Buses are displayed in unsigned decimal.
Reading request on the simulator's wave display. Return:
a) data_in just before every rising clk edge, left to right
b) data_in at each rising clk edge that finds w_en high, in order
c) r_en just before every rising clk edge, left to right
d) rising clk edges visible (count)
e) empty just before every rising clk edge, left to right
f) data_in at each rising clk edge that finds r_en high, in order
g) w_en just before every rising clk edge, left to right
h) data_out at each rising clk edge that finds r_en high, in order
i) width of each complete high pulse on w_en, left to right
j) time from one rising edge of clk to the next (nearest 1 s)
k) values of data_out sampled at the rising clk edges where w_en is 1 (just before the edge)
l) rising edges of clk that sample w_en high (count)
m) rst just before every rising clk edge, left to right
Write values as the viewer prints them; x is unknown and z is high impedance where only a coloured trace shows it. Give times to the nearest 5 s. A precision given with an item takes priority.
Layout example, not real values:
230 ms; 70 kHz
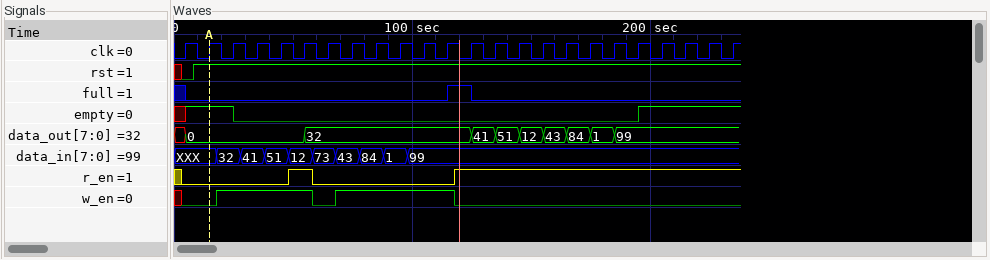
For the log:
XXX, XXX, 32, 41, 51, 12, 73, 43, 84, 1, 99, 99, 99, 99, 99, 99, 99, 99, 99, 99, 99, 99, 99, 99; 32, 41, 51, 12, 43, 84, 1, 99, 99; 0 0 0 0 0 1 0 0 0 0 0 0 1 1 1 1 1 1 1 1 1 1 1 1; 24; x 1 1 0 0 0 0 0 0 0 0 0 0 0 0 0 0 0 0 0 1 1 1 1; 12, 99, 99, 99, 99, 99, 99, 99, 99, 99, 99, 99, 99; 0 0 1 1 1 1 0 1 1 1 1 1 0 0 0 0 0 0 0 0 0 0 0 0; 0, 32, 41, 51, 12, 43, 84, 1, 99, 99, 99, 99, 99; 40 s, 50 s; 10 s; 0, 0, 0, 0, 32, 32, 32, 32, 32; 9; 0 1 1 1 1 1 1 1 1 1 1 1 1 1 1 1 1 1 1 1 1 1 1 1
